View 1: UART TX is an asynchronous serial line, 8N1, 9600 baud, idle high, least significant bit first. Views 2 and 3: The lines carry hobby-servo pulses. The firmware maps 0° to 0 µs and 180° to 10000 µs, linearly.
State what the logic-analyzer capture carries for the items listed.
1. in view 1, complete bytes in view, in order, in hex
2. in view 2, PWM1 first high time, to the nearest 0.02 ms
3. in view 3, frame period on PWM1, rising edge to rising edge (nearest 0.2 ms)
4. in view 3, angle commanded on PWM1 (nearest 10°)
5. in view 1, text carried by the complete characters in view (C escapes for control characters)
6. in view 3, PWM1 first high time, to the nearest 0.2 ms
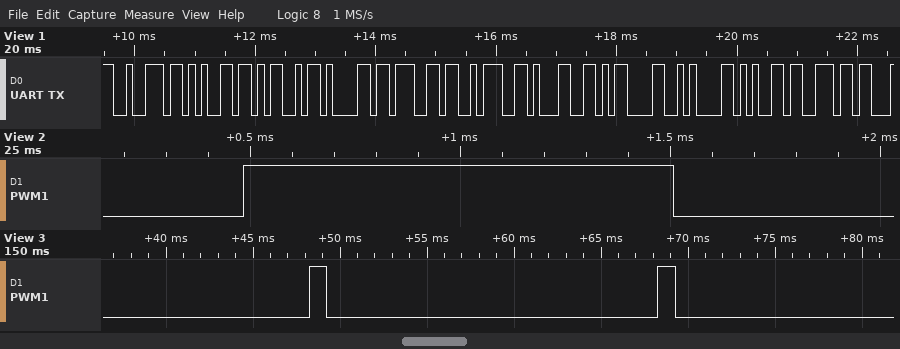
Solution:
72 65 4D 61 67 3A 31 0D 0A 65 6E
1.02 ms
20.0 ms
20°
"reMag:1\r\nen"
1.0 ms
